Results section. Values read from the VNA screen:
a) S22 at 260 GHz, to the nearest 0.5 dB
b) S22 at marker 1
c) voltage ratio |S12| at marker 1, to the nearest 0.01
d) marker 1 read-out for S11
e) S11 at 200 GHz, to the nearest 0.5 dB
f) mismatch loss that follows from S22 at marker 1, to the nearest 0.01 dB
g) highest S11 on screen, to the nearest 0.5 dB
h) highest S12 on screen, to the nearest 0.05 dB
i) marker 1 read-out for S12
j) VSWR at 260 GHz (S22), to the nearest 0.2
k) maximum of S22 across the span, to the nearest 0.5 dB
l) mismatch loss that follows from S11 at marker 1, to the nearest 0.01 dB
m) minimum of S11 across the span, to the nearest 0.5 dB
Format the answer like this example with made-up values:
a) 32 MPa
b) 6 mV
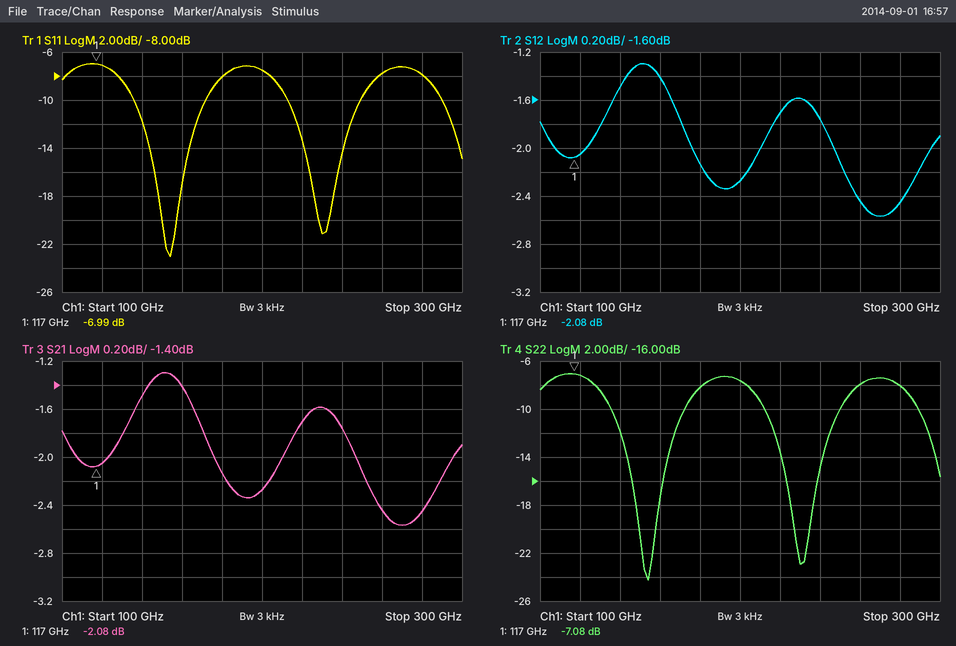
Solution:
a) -8.0 dB
b) -7.08 dB
c) 0.79
d) -6.99 dB
e) -7.5 dB
f) 0.95 dB
g) -7.0 dB
h) -1.30 dB
i) -2.08 dB
j) 2.4
k) -7.0 dB
l) 0.97 dB
m) -23.0 dB
